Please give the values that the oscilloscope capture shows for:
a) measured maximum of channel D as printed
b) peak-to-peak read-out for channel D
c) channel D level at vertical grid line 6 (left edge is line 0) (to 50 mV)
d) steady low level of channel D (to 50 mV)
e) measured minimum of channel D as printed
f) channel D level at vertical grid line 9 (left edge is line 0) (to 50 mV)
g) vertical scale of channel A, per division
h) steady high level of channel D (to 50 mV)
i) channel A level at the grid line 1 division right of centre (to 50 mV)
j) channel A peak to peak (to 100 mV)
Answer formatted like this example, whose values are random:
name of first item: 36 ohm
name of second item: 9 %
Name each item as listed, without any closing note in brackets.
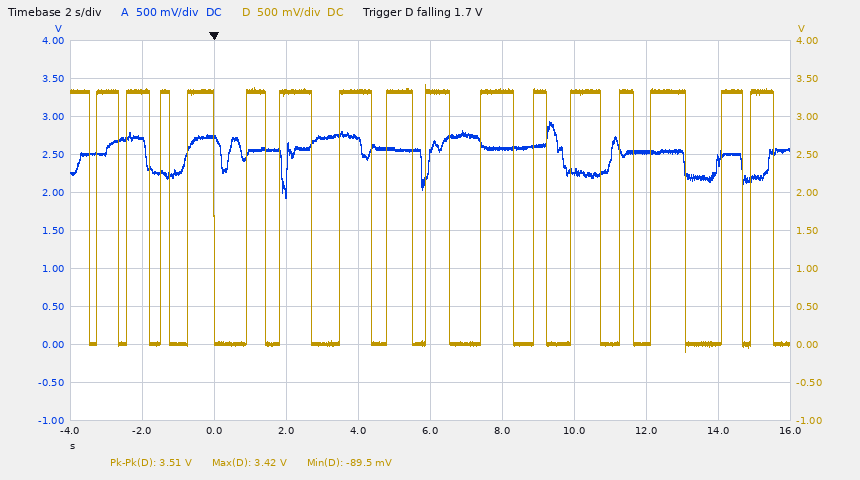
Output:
measured maximum of channel D as printed: 3.42 V
peak-to-peak read-out for channel D: 3.51 V
channel D level at vertical grid line 6 (left edge is line 0): 3.35 V
steady low level of channel D: 0 mV
measured minimum of channel D as printed: -89.5 mV
channel D level at vertical grid line 9 (left edge is line 0): 0 mV
vertical scale of channel A, per division: 500 mV
steady high level of channel D: 3.35 V
channel A level at the grid line 1 division right of centre: 2.60 V
channel A peak to peak: 1.00 V
